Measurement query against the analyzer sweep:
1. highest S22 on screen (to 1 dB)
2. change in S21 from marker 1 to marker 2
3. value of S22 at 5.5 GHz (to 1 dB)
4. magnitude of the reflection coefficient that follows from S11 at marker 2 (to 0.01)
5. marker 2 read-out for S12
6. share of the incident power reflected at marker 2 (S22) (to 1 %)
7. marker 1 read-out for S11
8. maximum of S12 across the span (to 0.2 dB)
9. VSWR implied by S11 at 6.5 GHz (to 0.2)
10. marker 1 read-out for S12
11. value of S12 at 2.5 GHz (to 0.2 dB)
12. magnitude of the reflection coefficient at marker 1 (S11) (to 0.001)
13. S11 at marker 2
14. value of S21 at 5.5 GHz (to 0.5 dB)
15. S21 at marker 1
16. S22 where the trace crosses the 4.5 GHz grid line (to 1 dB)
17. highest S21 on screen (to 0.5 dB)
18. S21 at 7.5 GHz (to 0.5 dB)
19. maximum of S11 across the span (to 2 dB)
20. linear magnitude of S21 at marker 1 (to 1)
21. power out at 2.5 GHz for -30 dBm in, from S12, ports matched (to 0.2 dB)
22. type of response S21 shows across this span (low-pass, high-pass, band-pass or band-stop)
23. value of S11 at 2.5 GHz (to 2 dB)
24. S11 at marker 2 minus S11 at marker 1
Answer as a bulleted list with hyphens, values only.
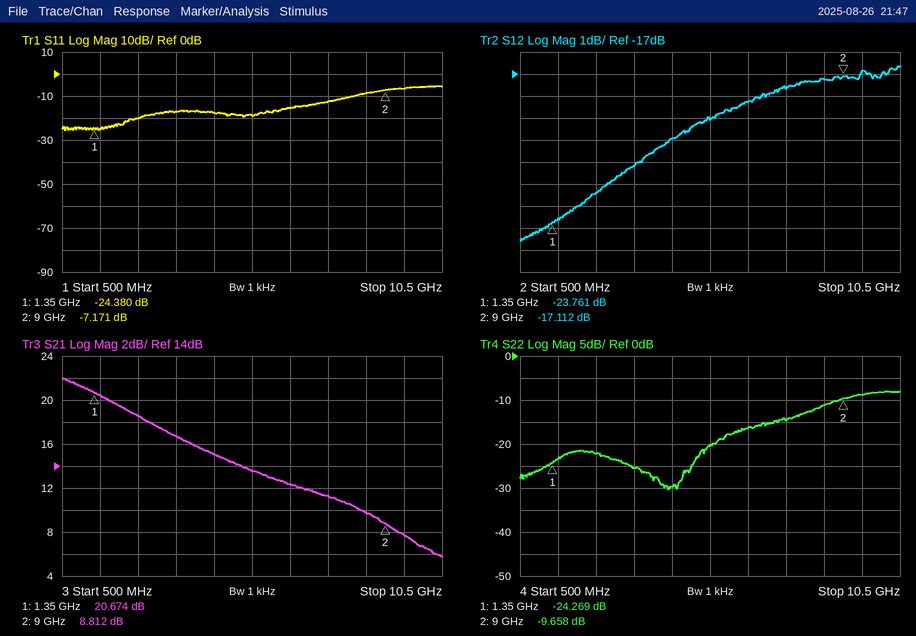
- -8 dB
- -11.862 dB
- -20 dB
- 0.44
- -17.112 dB
- 11 %
- -24.380 dB
- -16.6 dB
- 1.4
- -23.761 dB
- -22.4 dB
- 0.060
- -7.171 dB
- 13.5 dB
- 20.674 dB
- -30 dB
- 22.0 dB
- 11.5 dB
- -6 dB
- 11
- -52.4 dBm
- low-pass
- -20 dB
- 17.209 dB
